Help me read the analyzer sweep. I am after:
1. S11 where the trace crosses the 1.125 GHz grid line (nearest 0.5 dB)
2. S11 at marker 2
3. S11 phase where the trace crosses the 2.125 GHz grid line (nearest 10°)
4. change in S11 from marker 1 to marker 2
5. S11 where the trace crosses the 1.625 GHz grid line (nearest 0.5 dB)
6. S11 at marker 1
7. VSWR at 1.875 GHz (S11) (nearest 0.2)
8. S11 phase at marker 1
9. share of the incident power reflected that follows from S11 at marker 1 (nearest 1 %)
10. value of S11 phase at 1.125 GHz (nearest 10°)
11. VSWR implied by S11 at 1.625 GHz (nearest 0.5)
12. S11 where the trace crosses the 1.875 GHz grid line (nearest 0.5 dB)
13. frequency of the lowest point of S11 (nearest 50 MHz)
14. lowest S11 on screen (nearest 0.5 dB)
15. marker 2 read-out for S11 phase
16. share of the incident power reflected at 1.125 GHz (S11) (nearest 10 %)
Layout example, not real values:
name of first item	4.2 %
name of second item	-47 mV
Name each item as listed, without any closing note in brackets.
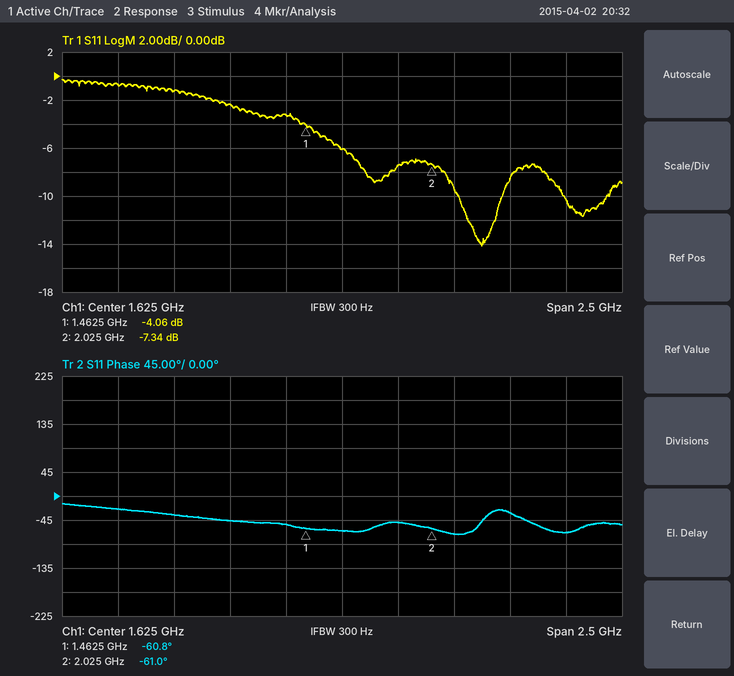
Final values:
S11 where the trace crosses the 1.125 GHz grid line	-2.5 dB
S11 at marker 2	-7.34 dB
S11 phase where the trace crosses the 2.125 GHz grid line	-70°
change in S11 from marker 1 to marker 2	-3.28 dB
S11 where the trace crosses the 1.625 GHz grid line	-6.0 dB
S11 at marker 1	-4.06 dB
VSWR at 1.875 GHz (S11)	2.4
S11 phase at marker 1	-60.8°
share of the incident power reflected that follows from S11 at marker 1	39 %
value of S11 phase at 1.125 GHz	-50°
VSWR implied by S11 at 1.625 GHz	3.0
S11 where the trace crosses the 1.875 GHz grid line	-7.5 dB
frequency of the lowest point of S11	2.25 GHz
lowest S11 on screen	-14.0 dB
marker 2 read-out for S11 phase	-61.0°
share of the incident power reflected at 1.125 GHz (S11)	60 %
